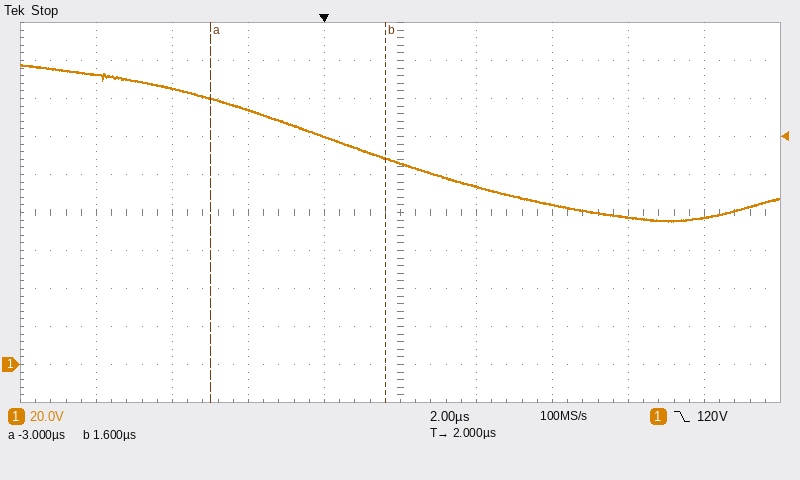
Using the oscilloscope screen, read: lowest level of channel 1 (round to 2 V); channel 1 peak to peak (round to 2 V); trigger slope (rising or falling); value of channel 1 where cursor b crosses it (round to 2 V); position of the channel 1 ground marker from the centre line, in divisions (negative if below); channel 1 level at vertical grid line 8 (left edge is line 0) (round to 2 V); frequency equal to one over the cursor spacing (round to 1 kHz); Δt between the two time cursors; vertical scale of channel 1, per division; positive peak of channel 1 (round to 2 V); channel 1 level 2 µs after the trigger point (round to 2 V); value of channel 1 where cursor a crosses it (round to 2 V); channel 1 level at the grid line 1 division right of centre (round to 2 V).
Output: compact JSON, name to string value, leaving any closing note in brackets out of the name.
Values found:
{"lowest level of channel 1": "76 V", "channel 1 peak to peak": "82 V", "trigger slope": "falling", "value of channel 1 where cursor b crosses it": "108 V", "position of the channel 1 ground marker from the centre line, in divisions": "-4.0 div", "channel 1 level at vertical grid line 8 (left edge is line 0)": "78 V", "frequency equal to one over the cursor spacing": "217 kHz", "Δt between the two time cursors": "4.6 µs", "vertical scale of channel 1, per division": "20 V", "positive peak of channel 1": "158 V", "channel 1 level 2 µs after the trigger point": "106 V", "value of channel 1 where cursor a crosses it": "140 V", "channel 1 level at the grid line 1 division right of centre": "94 V"}
